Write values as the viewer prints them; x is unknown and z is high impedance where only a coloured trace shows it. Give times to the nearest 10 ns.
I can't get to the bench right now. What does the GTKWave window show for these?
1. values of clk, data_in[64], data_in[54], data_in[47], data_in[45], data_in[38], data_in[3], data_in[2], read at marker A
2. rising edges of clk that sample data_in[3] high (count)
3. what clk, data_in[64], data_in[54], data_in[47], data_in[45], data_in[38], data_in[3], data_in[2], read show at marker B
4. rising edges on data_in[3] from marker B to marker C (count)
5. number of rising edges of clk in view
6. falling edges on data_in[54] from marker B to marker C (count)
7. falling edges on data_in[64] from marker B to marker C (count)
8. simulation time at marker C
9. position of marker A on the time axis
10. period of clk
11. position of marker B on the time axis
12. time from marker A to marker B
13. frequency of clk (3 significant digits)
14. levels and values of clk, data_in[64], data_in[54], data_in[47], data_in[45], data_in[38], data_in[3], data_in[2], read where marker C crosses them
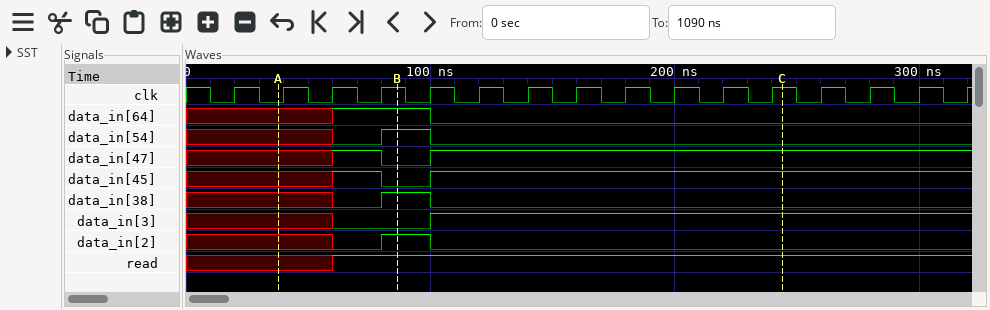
clk=0, data_in[64]=x, data_in[54]=x, data_in[47]=x, data_in[45]=x, data_in[38]=x, data_in[3]=x, data_in[2]=x, read=x
11
clk=1, data_in[64]=1, data_in[54]=1, data_in[47]=0, data_in[45]=0, data_in[38]=1, data_in[3]=0, data_in[2]=1, read=1
1
16
1
1
240 ns
40 ns
20 ns
90 ns
50 ns
50.0 MHz
clk=1, data_in[64]=0, data_in[54]=0, data_in[47]=1, data_in[45]=1, data_in[38]=0, data_in[3]=1, data_in[2]=0, read=1
